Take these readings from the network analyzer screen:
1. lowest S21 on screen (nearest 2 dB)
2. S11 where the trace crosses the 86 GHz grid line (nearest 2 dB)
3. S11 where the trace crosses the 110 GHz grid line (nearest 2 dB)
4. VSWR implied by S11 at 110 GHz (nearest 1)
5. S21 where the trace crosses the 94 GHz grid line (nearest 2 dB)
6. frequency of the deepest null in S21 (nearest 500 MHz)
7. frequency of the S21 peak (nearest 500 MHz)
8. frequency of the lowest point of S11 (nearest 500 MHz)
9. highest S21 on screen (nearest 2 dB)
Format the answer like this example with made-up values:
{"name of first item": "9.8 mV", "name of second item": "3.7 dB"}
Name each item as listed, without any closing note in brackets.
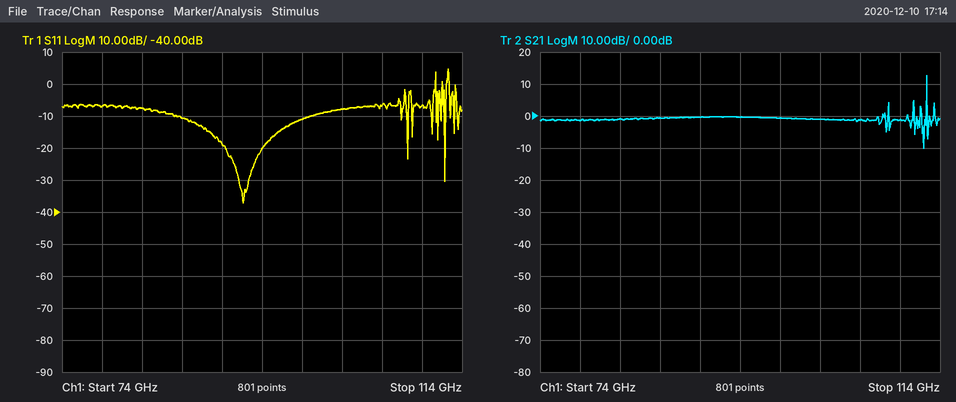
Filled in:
{"lowest S21 on screen": "-10 dB", "S11 where the trace crosses the 86 GHz grid line": "-10 dB", "S11 where the trace crosses the 110 GHz grid line": "-6 dB", "VSWR implied by S11 at 110 GHz": "3", "S21 where the trace crosses the 94 GHz grid line": "0 dB", "frequency of the deepest null in S21": "112.5 GHz", "frequency of the S21 peak": "112.5 GHz", "frequency of the lowest point of S11": "92.0 GHz", "highest S21 on screen": "12 dB"}
